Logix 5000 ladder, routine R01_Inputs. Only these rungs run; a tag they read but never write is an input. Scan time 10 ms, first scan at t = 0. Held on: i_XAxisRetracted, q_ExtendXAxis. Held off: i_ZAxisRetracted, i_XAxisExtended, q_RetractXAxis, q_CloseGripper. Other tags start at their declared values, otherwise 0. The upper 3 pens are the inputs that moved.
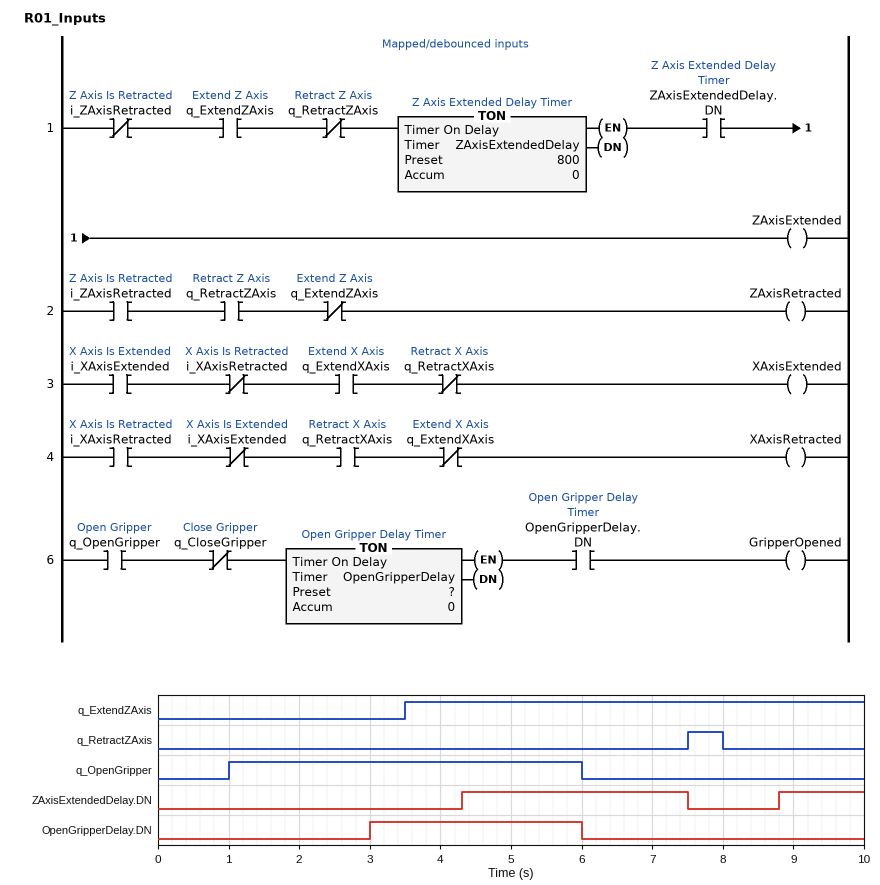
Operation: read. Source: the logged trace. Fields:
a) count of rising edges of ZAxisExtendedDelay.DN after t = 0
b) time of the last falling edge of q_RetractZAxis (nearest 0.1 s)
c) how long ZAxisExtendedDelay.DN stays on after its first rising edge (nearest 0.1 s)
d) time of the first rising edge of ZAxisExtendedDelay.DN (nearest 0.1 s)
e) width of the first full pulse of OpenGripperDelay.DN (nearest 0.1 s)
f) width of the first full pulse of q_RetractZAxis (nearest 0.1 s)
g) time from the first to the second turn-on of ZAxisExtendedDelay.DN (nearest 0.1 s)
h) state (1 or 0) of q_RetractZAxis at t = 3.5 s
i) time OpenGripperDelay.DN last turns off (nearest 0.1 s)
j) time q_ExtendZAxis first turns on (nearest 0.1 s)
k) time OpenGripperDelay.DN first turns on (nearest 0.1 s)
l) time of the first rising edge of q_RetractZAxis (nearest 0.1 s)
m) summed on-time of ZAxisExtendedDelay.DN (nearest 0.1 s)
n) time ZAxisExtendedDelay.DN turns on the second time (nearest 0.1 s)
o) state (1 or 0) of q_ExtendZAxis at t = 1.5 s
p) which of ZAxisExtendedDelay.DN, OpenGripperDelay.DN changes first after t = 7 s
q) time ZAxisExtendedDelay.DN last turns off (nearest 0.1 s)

2
8.0 s
3.2 s
4.3 s
3.0 s
0.5 s
4.5 s
0
6.0 s
3.5 s
3.0 s
7.5 s
4.4 s
8.8 s
0
ZAxisExtendedDelay.DN
7.5 s
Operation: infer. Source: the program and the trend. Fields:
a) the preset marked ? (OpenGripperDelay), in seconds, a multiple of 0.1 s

2.0 s
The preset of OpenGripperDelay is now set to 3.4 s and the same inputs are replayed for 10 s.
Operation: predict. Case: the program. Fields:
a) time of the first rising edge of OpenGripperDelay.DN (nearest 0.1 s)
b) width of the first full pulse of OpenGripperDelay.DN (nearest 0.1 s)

4.4 s
1.6 s
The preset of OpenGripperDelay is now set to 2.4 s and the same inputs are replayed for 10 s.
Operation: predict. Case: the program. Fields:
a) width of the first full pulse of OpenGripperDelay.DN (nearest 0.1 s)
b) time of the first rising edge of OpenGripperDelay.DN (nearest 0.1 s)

2.6 s
3.4 s
